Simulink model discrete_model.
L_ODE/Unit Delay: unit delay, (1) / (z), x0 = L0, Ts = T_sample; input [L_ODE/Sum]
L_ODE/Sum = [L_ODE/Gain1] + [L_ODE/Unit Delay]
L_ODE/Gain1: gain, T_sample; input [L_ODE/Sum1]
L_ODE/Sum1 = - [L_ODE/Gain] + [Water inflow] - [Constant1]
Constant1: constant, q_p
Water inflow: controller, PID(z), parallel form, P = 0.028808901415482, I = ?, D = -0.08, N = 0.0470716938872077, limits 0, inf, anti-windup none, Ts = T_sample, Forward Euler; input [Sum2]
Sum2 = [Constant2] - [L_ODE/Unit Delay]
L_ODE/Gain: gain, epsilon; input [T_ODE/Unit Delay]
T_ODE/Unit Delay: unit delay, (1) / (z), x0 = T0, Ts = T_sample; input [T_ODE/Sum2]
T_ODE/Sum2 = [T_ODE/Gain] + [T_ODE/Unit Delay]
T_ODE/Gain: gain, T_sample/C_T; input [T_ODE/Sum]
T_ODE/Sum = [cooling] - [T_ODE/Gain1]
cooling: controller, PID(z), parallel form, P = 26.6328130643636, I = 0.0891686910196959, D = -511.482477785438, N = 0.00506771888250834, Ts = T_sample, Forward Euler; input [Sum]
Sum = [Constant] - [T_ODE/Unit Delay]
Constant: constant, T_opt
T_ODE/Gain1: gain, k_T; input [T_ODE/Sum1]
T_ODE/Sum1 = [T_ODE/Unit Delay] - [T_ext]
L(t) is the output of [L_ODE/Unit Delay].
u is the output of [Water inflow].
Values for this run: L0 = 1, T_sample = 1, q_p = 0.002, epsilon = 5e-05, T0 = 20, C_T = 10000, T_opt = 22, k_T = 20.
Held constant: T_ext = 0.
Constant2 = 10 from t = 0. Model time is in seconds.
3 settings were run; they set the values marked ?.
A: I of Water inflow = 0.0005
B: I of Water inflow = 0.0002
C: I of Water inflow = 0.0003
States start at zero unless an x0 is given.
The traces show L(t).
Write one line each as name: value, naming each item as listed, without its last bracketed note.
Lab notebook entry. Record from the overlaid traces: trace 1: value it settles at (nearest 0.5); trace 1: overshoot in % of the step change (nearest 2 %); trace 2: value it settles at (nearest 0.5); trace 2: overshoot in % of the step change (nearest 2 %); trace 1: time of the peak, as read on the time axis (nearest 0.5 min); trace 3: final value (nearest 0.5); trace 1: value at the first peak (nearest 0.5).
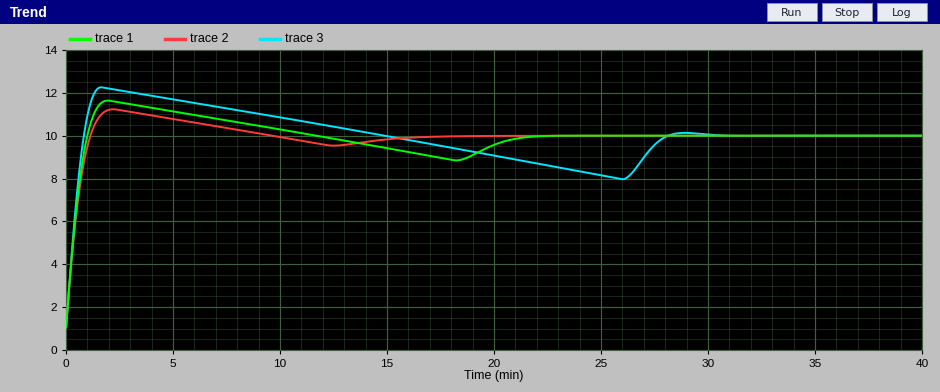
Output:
trace 1: value it settles at: 10.0
trace 1: overshoot in % of the step change: 18 %
trace 2: value it settles at: 10.0
trace 2: overshoot in % of the step change: 14 %
trace 1: time of the peak, as read on the time axis: 2.0 min
trace 3: final value: 10.0
trace 1: value at the first peak: 11.5
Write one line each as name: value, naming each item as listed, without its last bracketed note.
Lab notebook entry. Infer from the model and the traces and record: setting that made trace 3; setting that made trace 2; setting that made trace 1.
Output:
setting that made trace 3: A
setting that made trace 2: B
setting that made trace 1: C
